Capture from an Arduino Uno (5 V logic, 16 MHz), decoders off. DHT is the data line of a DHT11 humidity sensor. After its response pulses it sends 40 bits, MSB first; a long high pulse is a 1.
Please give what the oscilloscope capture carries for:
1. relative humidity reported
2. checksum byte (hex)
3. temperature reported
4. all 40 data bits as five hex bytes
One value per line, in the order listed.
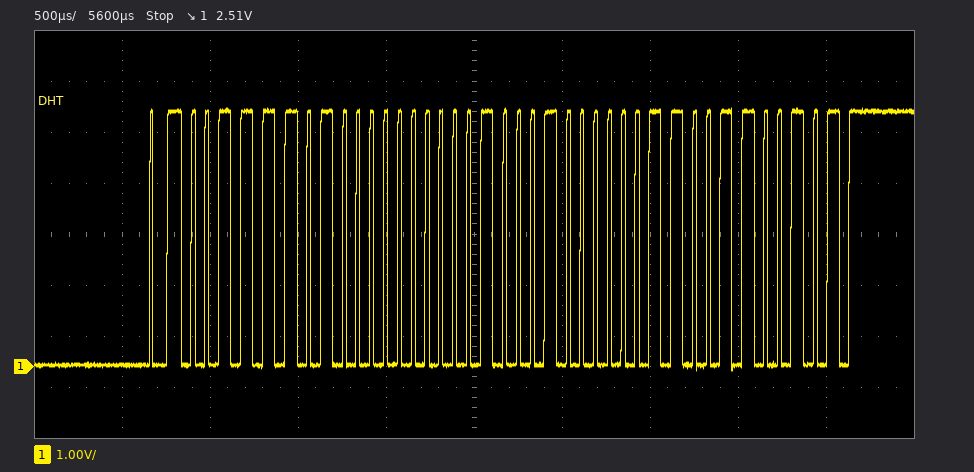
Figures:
61 %
0x65
34.6 °C
3D 00 22 06 65
